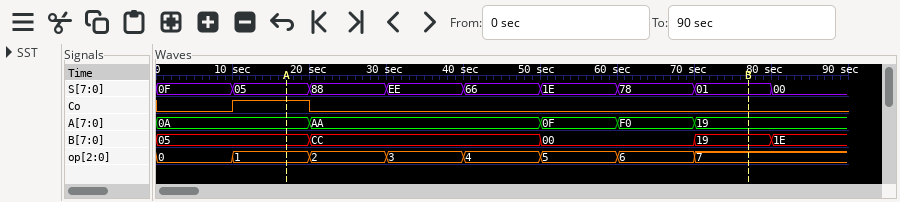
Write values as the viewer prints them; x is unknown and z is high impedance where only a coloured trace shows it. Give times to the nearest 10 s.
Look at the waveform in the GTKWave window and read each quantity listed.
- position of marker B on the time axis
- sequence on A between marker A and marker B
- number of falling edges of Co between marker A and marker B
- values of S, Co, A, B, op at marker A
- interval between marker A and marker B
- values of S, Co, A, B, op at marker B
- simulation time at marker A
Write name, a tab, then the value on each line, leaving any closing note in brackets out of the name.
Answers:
position of marker B on the time axis	80 s
sequence on A between marker A and marker B	0A, AA, 0F, F0, 19
number of falling edges of Co between marker A and marker B	1
values of S, Co, A, B, op at marker A	S=05, Co=1, A=0A, B=05, op=1
interval between marker A and marker B	60 s
values of S, Co, A, B, op at marker B	S=01, Co=0, A=19, B=19, op=7
simulation time at marker A	20 s
